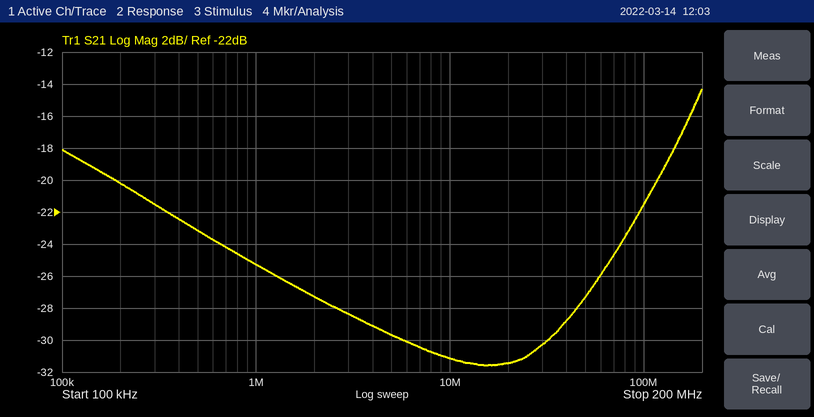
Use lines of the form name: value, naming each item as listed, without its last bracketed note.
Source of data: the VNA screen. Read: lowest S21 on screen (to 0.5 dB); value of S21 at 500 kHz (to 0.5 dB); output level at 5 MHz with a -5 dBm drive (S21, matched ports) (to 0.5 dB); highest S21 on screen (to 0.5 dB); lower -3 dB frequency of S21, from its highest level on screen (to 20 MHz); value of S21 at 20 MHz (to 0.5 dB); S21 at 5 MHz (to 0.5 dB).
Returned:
lowest S21 on screen: -31.5 dB
value of S21 at 500 kHz: -23.0 dB
output level at 5 MHz with a -5 dBm drive (S21, matched ports): -34.5 dBm
highest S21 on screen: -14.5 dB
lower -3 dB frequency of S21, from its highest level on screen: 160 MHz
value of S21 at 20 MHz: -31.5 dB
S21 at 5 MHz: -29.5 dB
